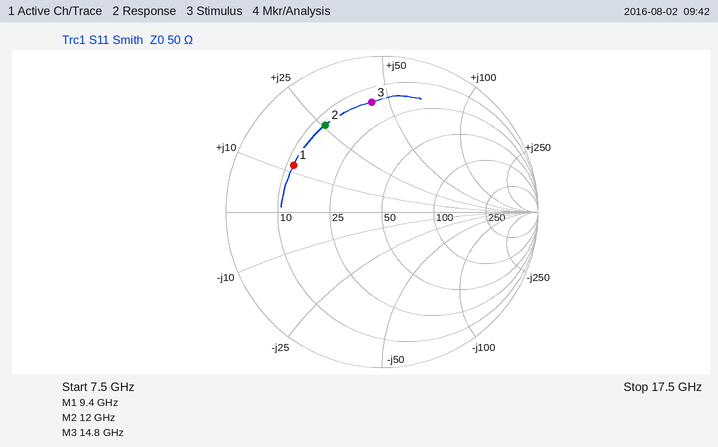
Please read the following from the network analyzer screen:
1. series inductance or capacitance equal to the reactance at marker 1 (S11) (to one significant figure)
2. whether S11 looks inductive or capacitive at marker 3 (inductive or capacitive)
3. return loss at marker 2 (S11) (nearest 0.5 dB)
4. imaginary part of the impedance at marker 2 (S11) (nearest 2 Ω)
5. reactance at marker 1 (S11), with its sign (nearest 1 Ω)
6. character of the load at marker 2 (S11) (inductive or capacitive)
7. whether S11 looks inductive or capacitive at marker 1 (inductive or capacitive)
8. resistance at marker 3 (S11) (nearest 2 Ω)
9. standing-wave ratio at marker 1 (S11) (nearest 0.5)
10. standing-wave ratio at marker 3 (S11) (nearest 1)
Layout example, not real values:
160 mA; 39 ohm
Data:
200 pH; inductive; 3.5 dB; +26 Ω; +12 Ω; inductive; inductive; 16 Ω; 4.5; 6
